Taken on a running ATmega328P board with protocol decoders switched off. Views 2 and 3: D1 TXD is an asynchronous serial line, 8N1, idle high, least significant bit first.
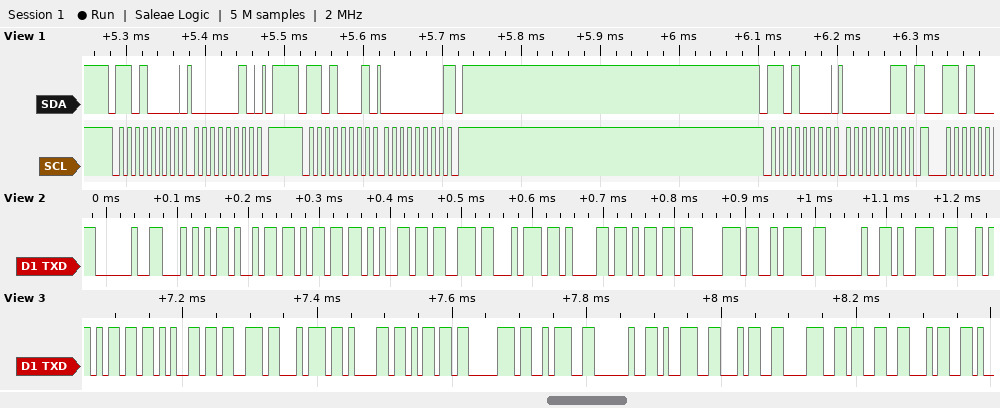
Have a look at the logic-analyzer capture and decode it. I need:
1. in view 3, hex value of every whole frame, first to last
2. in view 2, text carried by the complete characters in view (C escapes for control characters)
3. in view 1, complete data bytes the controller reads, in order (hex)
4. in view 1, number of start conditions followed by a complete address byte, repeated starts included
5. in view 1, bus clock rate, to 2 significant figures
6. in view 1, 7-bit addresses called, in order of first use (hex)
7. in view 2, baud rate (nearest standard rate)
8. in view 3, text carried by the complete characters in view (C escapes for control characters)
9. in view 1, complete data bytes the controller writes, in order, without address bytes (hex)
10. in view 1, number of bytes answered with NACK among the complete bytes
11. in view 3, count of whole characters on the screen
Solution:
6D 65 73 74 61 6D 70 3A 20 39 34 38 33 34
" Timestamp: 9"
00
3
100 kHz
0x68
115200 baud
"mestamp: 94834"
02 03
1
14
